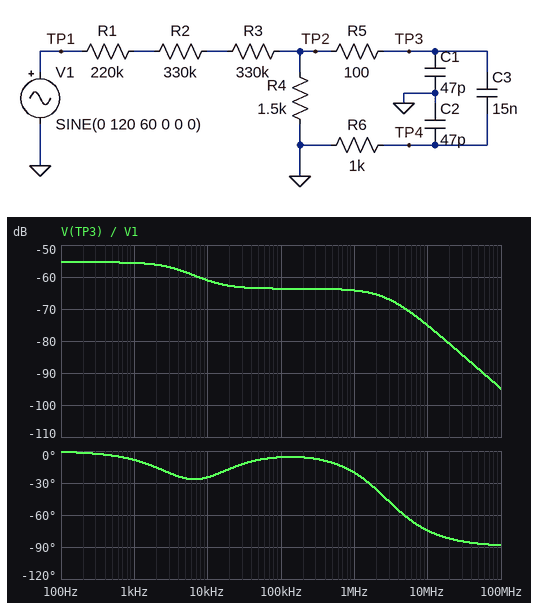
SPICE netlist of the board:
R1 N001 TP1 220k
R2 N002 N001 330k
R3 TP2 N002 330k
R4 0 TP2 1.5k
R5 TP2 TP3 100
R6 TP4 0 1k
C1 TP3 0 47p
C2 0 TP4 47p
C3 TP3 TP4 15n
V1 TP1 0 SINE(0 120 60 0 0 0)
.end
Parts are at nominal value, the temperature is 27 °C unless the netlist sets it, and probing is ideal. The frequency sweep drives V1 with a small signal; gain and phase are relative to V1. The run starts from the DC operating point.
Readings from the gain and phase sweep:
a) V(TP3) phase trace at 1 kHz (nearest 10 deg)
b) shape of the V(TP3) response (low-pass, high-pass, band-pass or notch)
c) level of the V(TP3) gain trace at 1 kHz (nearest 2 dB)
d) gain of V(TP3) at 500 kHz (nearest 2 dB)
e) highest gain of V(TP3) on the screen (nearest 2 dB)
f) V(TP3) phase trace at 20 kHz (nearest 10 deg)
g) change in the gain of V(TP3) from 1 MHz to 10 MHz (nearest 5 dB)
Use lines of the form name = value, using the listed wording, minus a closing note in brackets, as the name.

V(TP3) phase trace at 1 kHz = -10 deg
shape of the V(TP3) response = low-pass
level of the V(TP3) gain trace at 1 kHz = -56 dB
gain of V(TP3) at 500 kHz = -64 dB
highest gain of V(TP3) on the screen = -56 dB
V(TP3) phase trace at 20 kHz = -20 deg
change in the gain of V(TP3) from 1 MHz to 10 MHz = -10 dB
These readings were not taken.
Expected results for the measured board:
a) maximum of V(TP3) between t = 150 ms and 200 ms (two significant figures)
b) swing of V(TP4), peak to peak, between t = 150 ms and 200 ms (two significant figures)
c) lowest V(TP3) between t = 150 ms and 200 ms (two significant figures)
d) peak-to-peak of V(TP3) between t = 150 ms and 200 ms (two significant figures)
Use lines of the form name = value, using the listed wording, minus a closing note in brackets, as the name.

maximum of V(TP3) between t = 150 ms and 200 ms = 200 mV
swing of V(TP4), peak to peak, between t = 150 ms and 200 ms = 2.3 mV
lowest V(TP3) between t = 150 ms and 200 ms = -200 mV
peak-to-peak of V(TP3) between t = 150 ms and 200 ms = 410 mV
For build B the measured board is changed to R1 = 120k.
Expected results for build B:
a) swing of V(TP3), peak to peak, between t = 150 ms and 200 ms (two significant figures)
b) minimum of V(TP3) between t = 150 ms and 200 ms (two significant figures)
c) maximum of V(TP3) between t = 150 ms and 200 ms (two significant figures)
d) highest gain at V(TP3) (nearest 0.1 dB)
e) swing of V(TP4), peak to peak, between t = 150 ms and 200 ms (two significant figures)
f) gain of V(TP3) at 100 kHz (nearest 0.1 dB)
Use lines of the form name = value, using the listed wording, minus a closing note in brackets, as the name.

swing of V(TP3), peak to peak, between t = 150 ms and 200 ms = 460 mV
minimum of V(TP3) between t = 150 ms and 200 ms = -230 mV
maximum of V(TP3) between t = 150 ms and 200 ms = 230 mV
highest gain at V(TP3) = -54.3 dB
swing of V(TP4), peak to peak, between t = 150 ms and 200 ms = 2.6 mV
gain of V(TP3) at 100 kHz = -62.6 dB
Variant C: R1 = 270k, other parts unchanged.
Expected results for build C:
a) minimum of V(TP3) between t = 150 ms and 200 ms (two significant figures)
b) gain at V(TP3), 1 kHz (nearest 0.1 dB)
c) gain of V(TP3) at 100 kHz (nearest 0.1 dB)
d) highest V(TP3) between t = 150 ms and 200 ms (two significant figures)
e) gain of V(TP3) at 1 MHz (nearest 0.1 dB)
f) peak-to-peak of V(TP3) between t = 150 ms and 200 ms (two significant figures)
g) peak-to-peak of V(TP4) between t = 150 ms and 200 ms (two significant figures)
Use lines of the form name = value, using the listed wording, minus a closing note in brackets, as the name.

minimum of V(TP3) between t = 150 ms and 200 ms = -190 mV
gain at V(TP3), 1 kHz = -56.1 dB
gain of V(TP3) at 100 kHz = -64.1 dB
highest V(TP3) between t = 150 ms and 200 ms = 190 mV
gain of V(TP3) at 1 MHz = -64.7 dB
peak-to-peak of V(TP3) between t = 150 ms and 200 ms = 390 mV
peak-to-peak of V(TP4) between t = 150 ms and 200 ms = 2.2 mV
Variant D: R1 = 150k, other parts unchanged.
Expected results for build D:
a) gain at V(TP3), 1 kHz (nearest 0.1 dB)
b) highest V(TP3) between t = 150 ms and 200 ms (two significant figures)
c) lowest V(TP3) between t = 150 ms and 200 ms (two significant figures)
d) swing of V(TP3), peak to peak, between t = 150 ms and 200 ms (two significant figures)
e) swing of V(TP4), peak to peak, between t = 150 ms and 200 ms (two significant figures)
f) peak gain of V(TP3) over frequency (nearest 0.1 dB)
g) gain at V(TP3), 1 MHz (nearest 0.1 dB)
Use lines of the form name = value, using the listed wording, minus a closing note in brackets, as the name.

gain at V(TP3), 1 kHz = -54.9 dB
highest V(TP3) between t = 150 ms and 200 ms = 220 mV
lowest V(TP3) between t = 150 ms and 200 ms = -220 mV
swing of V(TP3), peak to peak, between t = 150 ms and 200 ms = 440 mV
swing of V(TP4), peak to peak, between t = 150 ms and 200 ms = 2.5 mV
peak gain of V(TP3) over frequency = -54.7 dB
gain at V(TP3), 1 MHz = -63.5 dB
